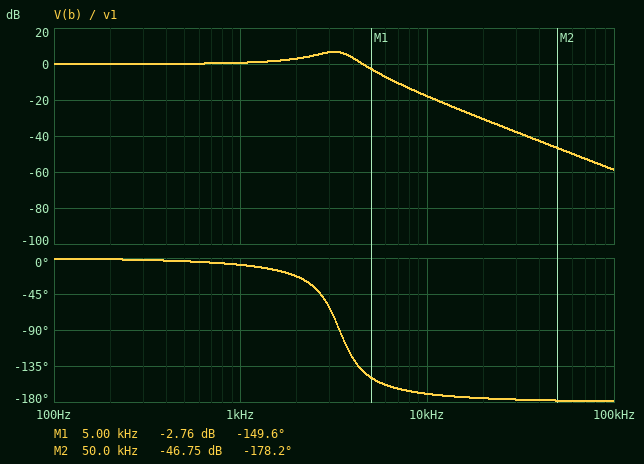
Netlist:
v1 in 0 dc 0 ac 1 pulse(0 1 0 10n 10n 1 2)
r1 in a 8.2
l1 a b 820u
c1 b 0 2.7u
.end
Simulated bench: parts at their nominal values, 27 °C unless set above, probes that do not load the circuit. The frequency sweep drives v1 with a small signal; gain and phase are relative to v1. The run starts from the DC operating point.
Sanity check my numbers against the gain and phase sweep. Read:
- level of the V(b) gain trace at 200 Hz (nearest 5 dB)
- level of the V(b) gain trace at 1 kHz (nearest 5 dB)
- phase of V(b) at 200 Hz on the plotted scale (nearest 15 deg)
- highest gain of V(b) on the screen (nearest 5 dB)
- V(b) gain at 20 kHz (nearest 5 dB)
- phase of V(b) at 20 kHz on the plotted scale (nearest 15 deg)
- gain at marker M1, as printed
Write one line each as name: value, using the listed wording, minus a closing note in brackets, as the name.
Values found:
level of the V(b) gain trace at 200 Hz: 0 dB
level of the V(b) gain trace at 1 kHz: 0 dB
phase of V(b) at 200 Hz on the plotted scale: 0 deg
highest gain of V(b) on the screen: 5 dB
V(b) gain at 20 kHz: -30 dB
phase of V(b) at 20 kHz on the plotted scale: -180 deg
gain at marker M1, as printed: -2.76 dB
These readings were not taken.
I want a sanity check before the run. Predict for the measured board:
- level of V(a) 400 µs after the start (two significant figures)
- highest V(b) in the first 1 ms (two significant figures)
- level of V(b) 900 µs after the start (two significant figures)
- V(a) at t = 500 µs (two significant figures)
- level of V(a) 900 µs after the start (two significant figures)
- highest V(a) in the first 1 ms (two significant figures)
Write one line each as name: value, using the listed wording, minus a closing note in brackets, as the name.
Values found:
level of V(a) 400 µs after the start: 940 mV
highest V(b) in the first 1 ms: 1.5 V
level of V(b) 900 µs after the start: 990 mV
V(a) at t = 500 µs: 1.0 V
level of V(a) 900 µs after the start: 1.0 V
highest V(a) in the first 1 ms: 1.2 V
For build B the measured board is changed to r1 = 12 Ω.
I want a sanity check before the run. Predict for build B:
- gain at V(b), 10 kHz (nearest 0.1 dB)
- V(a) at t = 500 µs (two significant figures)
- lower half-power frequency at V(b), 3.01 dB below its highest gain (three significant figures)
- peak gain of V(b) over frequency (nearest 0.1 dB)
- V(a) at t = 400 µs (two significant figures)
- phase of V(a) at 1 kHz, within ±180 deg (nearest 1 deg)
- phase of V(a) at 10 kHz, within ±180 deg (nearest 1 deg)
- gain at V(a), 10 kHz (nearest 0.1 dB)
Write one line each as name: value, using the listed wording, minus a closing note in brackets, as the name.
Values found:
gain at V(b), 10 kHz: -18.1 dB
V(a) at t = 500 µs: 1.0 V
lower half-power frequency at V(b), 3.01 dB below its highest gain: 1.15 kHz
peak gain of V(b) over frequency: 3.8 dB
V(a) at t = 400 µs: 960 mV
phase of V(a) at 1 kHz, within ±180 deg: -13 deg
phase of V(a) at 10 kHz, within ±180 deg: 15 deg
gain at V(a), 10 kHz: -0.3 dB
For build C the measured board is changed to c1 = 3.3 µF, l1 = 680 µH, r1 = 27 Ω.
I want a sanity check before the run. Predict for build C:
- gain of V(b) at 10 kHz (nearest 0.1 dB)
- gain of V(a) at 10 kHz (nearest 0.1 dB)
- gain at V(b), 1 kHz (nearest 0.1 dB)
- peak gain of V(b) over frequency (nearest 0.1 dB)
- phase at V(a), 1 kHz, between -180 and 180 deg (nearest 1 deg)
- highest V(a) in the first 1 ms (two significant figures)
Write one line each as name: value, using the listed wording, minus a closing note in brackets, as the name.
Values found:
gain of V(b) at 10 kHz: -19.7 dB
gain of V(a) at 10 kHz: -1.8 dB
gain at V(b), 1 kHz: -0.6 dB
peak gain of V(b) over frequency: 0 dB
phase at V(a), 1 kHz, between -180 and 180 deg: -32 deg
highest V(a) in the first 1 ms: 1.0 V
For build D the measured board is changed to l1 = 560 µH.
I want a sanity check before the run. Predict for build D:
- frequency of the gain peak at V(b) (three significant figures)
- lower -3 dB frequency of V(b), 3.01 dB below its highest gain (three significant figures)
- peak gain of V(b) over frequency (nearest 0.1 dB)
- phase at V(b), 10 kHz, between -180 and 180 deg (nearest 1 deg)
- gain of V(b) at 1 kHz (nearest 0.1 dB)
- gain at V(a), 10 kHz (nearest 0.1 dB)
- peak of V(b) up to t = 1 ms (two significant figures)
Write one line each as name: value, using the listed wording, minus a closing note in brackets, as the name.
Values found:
frequency of the gain peak at V(b): 3.75 kHz
lower -3 dB frequency of V(b), 3.01 dB below its highest gain: 2.21 kHz
peak gain of V(b) over frequency: 5.3 dB
phase at V(b), 10 kHz, between -180 and 180 deg: -164 deg
gain of V(b) at 1 kHz: 0.4 dB
gain at V(a), 10 kHz: -0.3 dB
peak of V(b) up to t = 1 ms: 1.4 V
